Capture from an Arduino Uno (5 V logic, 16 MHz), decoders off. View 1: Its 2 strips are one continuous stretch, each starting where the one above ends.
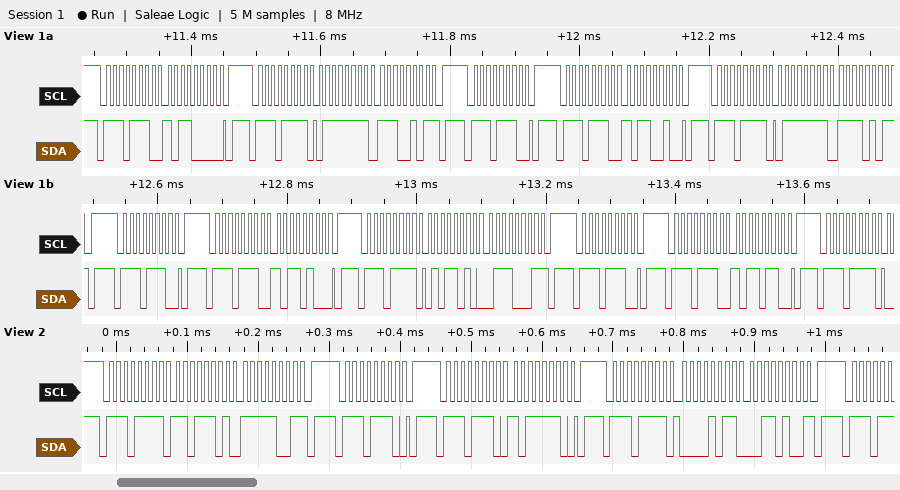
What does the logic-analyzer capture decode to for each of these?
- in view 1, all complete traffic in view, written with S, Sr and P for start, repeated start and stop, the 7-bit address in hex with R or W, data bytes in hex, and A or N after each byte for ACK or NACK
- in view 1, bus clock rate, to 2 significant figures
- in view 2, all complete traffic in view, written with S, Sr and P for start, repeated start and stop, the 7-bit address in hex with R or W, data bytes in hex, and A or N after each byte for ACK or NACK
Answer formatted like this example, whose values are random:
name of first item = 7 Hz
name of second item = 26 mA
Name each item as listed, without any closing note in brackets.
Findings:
in view 1, all complete traffic in view, written with S, Sr and P for start, repeated start and stop, the 7-bit address in hex with R or W, data bytes in hex, and A or N after each byte for ACK or NACK = S 77W A B0 A P S 77R A 7F A E5 N P S 77W A P S 77W A B2 A P S 77R A 7F A F5 N P S 77W A P S 77W A B4 A P S 77R A 5A A 71 N P S 77W A P S 77W A B6 A P S 77R A
in view 1, bus clock rate, to 2 significant figures = 100 kHz
in view 2, all complete traffic in view, written with S, Sr and P for start, repeated start and stop, the 7-bit address in hex with R or W, data bytes in hex, and A or N after each byte for ACK or NACK = S 77R A DD A F9 N P S 77W A P S 77W A BE A P S 77R A 0B A 34 N P
